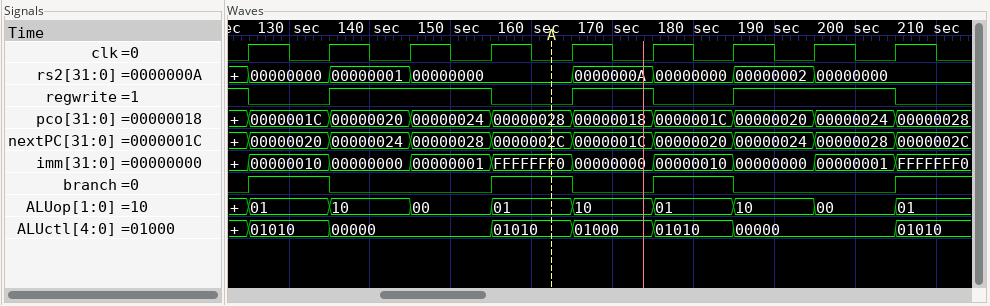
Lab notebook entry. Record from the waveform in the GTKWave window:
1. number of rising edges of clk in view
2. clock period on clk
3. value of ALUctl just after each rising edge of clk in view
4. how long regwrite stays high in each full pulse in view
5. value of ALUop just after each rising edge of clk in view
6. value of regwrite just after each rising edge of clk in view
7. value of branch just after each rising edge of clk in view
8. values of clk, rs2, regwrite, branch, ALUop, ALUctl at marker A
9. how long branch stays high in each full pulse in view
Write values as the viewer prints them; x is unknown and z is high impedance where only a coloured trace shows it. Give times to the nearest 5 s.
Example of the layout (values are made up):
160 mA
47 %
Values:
9
10 s
01010, 00000, 00000, 01010, 01000, 01010, 00000, 00000, 01010
20 s, 10 s, 20 s
01, 10, 00, 01, 10, 01, 10, 00, 01
0 1 1 0 1 0 1 1 0
1 0 0 1 0 1 0 0 1
clk=0, rs2=00000000, regwrite=0, branch=1, ALUop=01, ALUctl=01010
10 s, 10 s, 10 s
